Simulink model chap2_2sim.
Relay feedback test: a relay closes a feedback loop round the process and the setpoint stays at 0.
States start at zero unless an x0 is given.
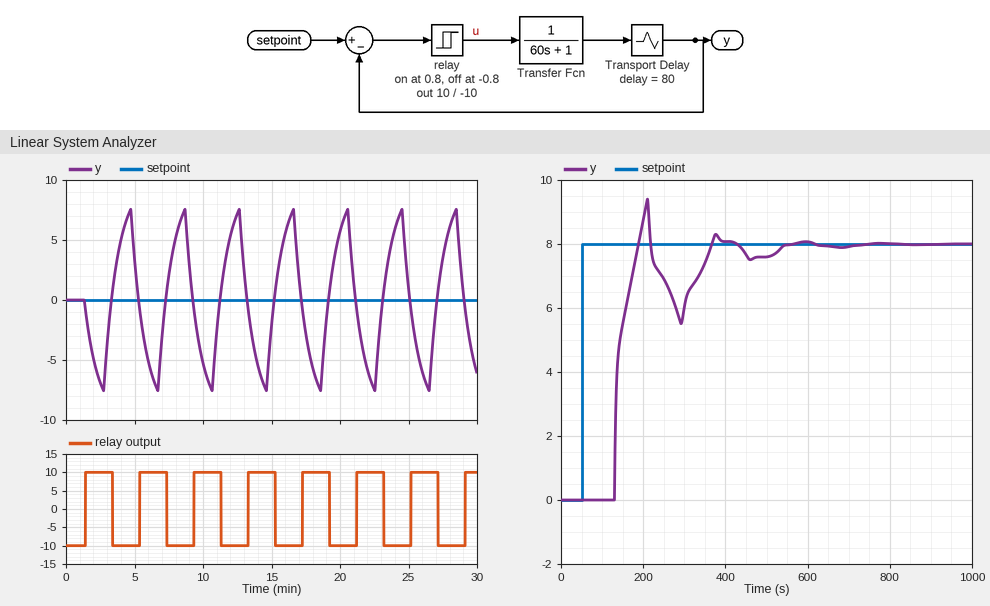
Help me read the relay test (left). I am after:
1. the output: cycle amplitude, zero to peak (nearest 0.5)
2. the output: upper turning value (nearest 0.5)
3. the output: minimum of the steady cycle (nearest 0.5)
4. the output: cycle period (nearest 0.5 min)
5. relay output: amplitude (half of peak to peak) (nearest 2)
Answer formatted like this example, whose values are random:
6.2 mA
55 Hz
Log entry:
7.5
7.5
-7.5
4.0 min
10
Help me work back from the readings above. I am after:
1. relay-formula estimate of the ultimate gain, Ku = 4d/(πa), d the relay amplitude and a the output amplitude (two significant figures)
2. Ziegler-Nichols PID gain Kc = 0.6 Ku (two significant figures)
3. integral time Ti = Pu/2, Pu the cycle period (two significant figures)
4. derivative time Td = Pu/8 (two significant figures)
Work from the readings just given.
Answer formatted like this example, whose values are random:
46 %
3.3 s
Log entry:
1.7
1.0
2.0 min
0.50 min
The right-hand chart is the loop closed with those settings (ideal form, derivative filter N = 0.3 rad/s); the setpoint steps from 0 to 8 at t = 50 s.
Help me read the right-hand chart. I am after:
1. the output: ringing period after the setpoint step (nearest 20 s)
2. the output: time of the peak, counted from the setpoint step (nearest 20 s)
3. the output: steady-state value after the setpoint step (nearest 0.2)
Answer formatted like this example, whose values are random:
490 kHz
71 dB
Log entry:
160 s
160 s
8.0
